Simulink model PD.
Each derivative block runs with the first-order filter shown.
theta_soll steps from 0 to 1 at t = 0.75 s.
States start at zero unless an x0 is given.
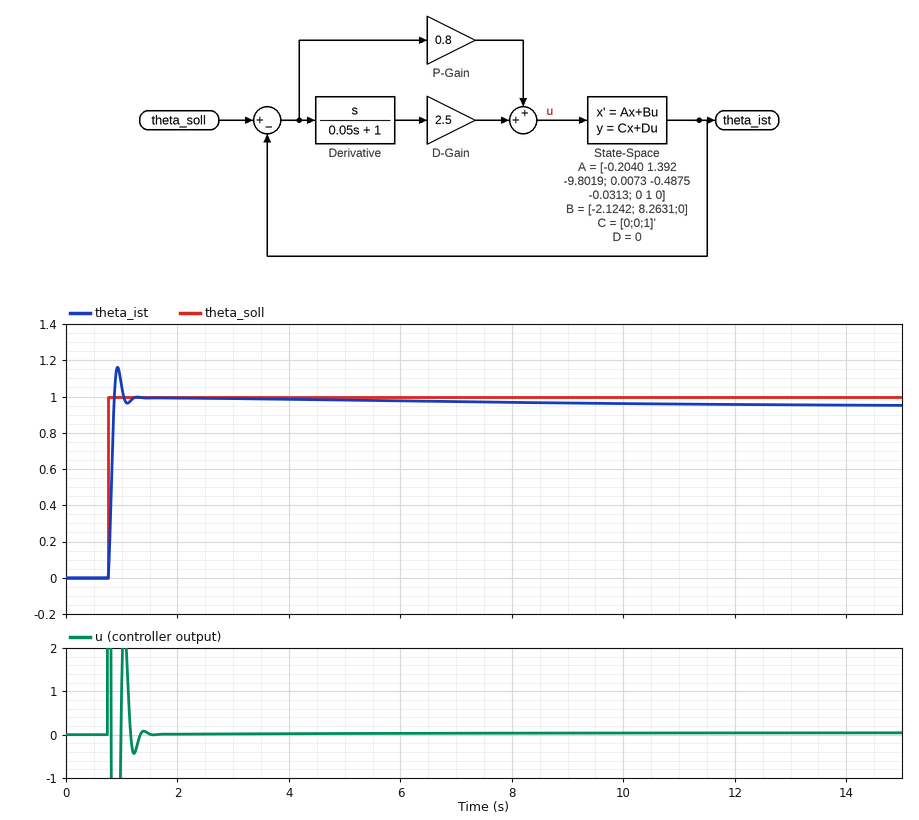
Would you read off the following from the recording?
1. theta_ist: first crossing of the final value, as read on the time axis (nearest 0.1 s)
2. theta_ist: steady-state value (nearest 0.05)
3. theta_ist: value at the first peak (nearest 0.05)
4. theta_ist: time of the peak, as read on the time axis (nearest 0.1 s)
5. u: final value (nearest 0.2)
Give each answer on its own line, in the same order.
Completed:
0.9 s
0.95
1.15
0.9 s
0.0
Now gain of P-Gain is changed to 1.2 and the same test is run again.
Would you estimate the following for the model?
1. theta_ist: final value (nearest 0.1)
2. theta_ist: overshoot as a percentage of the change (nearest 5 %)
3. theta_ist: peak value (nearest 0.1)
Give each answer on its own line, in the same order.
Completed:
1.0
20 %
1.2
